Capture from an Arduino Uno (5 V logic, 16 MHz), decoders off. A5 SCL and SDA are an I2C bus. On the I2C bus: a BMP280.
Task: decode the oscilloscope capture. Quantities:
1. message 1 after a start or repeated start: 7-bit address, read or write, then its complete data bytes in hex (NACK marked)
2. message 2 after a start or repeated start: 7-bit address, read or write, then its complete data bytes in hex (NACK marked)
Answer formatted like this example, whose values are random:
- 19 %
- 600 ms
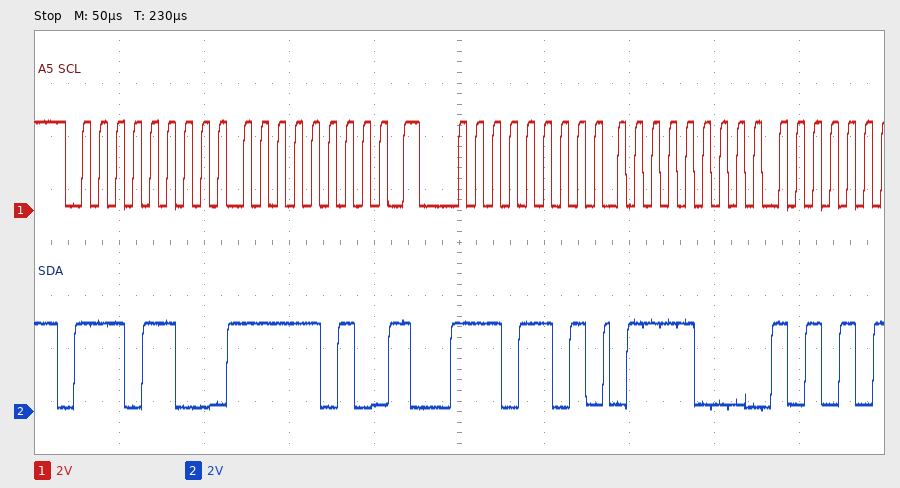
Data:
- 0x76 write: FA
- 0x76 read: 78
